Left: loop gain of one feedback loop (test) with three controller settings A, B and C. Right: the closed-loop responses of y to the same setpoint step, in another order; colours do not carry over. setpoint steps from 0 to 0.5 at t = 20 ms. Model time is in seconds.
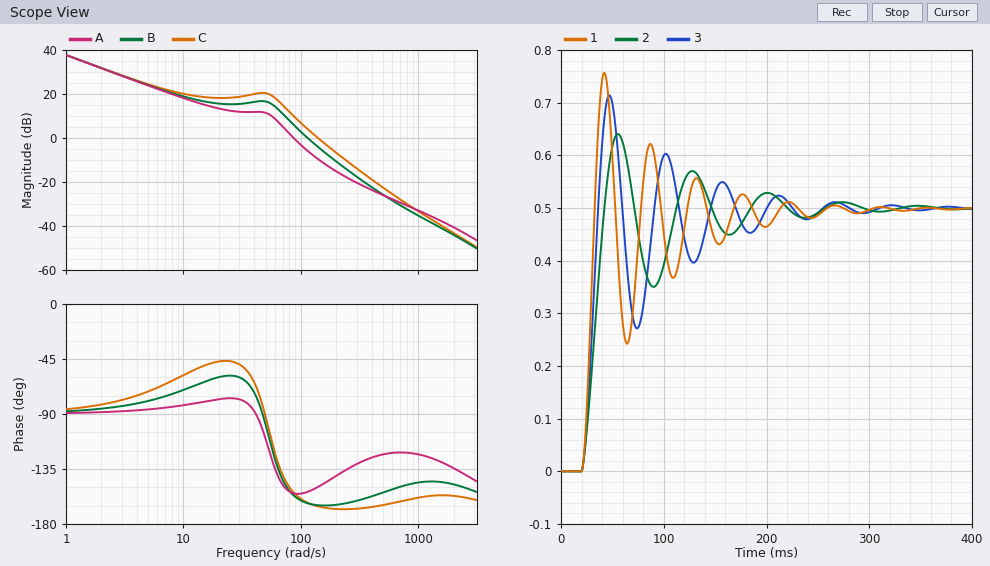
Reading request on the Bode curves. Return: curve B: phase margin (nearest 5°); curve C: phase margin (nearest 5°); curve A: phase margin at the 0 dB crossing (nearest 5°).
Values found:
15°
15°
25°
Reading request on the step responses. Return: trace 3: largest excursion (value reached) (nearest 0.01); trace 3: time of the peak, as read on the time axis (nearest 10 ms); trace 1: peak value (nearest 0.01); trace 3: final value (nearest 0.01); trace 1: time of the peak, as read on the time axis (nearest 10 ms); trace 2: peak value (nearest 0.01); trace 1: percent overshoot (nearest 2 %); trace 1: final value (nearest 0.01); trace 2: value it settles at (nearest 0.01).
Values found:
0.71
50 ms
0.76
0.50
40 ms
0.64
52 %
0.50
0.50
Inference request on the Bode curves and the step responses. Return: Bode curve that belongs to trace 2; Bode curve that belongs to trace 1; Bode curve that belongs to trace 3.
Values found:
A
C
B
